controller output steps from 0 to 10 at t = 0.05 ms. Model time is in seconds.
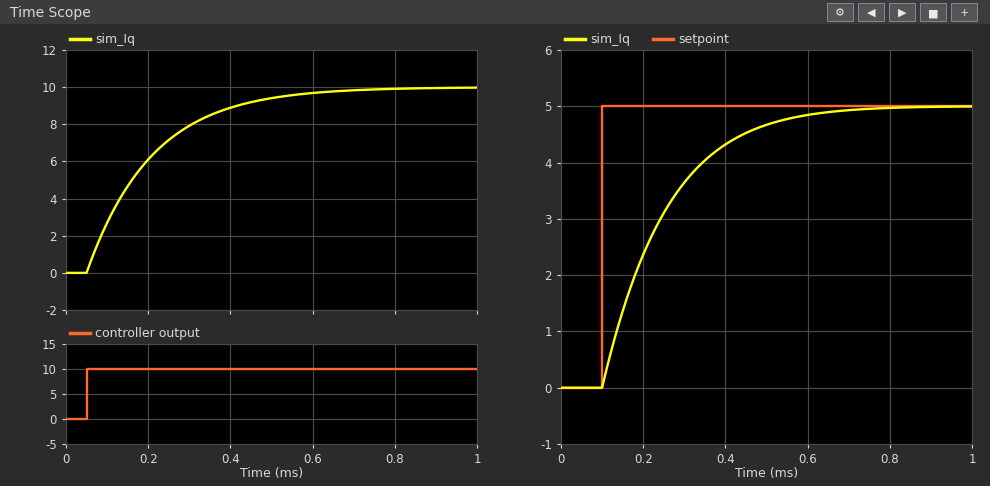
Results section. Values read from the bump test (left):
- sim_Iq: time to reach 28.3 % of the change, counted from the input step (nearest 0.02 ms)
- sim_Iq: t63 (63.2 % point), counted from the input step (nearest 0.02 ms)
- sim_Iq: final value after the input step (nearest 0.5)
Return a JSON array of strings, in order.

["0.06 ms", "0.16 ms", "10.0"]
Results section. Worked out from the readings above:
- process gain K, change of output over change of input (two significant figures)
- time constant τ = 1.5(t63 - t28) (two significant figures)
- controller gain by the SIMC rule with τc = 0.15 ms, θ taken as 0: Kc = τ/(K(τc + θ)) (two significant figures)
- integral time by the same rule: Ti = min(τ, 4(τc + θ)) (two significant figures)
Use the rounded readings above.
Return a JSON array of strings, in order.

["1.0", "0.15 ms", "1.0", "0.15 ms"]
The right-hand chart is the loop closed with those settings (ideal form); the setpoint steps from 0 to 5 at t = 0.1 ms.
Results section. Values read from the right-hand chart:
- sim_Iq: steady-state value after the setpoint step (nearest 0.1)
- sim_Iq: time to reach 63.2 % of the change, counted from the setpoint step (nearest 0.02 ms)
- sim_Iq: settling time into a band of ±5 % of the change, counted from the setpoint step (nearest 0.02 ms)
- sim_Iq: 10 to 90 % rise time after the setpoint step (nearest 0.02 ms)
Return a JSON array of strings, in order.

["5.0", "0.16 ms", "0.44 ms", "0.32 ms"]
